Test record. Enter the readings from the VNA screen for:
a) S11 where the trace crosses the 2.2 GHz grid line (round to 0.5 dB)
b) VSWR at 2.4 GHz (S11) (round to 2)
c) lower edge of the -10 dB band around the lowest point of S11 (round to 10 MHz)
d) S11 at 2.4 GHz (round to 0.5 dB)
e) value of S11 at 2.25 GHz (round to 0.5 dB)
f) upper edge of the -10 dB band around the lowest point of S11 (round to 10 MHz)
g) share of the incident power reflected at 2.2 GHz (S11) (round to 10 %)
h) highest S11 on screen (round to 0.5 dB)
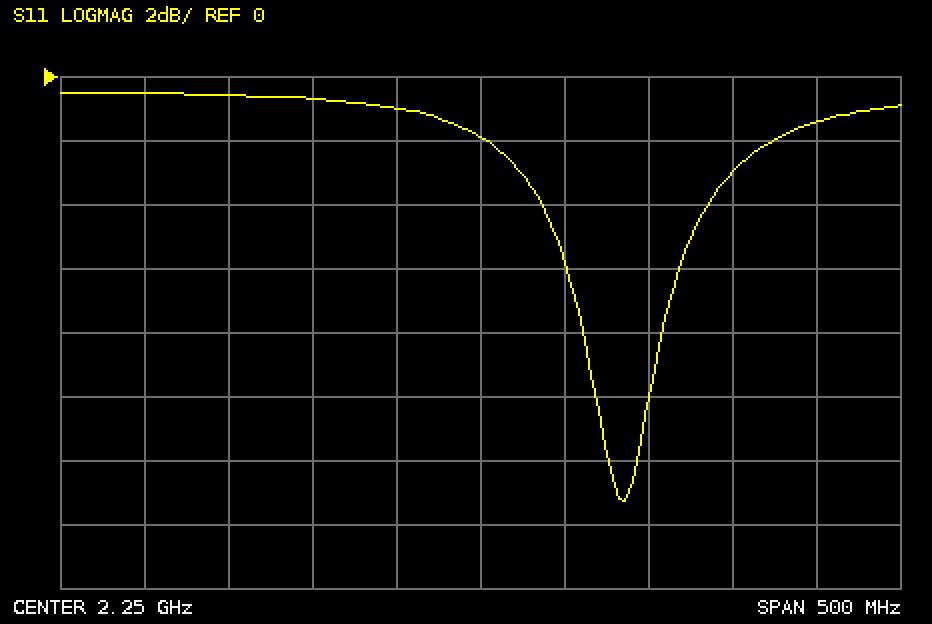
-1.0 dB
6
2.32 GHz
-3.0 dB
-2.0 dB
2.35 GHz
80 %
-0.5 dB
